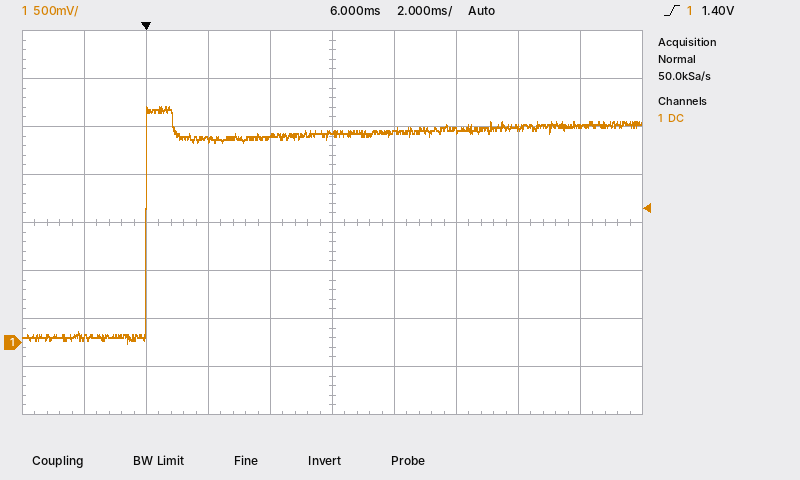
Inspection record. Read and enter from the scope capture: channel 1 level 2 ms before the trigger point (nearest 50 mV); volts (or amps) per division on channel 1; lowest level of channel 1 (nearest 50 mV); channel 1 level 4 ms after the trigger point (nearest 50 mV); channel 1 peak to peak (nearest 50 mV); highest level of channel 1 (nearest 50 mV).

50 mV
500 mV
0 mV
2.15 V
2.45 V
2.45 V
